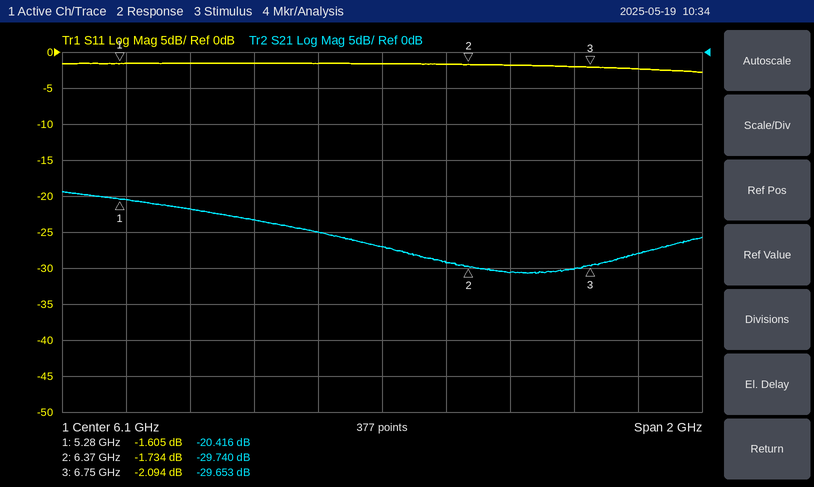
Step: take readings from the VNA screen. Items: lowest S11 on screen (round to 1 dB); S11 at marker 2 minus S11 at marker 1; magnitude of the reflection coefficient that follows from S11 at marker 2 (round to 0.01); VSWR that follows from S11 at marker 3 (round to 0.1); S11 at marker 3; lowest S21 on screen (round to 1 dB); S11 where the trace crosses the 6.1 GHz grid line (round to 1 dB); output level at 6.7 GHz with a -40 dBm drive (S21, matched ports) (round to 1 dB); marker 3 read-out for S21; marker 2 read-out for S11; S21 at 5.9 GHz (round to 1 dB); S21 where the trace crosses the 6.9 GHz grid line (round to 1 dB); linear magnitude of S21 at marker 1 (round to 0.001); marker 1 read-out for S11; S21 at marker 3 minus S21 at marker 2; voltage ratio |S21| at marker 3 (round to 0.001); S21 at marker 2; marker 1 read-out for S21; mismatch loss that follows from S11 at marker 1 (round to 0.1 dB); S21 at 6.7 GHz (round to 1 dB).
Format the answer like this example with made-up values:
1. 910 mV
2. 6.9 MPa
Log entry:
1. -3 dB
2. -0.129 dB
3. 0.82
4. 8.3
5. -2.094 dB
6. -31 dB
7. -2 dB
8. -70 dBm
9. -29.653 dB
10. -1.734 dB
11. -25 dB
12. -28 dB
13. 0.095
14. -1.605 dB
15. 0.087 dB
16. 0.033
17. -29.740 dB
18. -20.416 dB
19. 5.1 dB
20. -30 dB
